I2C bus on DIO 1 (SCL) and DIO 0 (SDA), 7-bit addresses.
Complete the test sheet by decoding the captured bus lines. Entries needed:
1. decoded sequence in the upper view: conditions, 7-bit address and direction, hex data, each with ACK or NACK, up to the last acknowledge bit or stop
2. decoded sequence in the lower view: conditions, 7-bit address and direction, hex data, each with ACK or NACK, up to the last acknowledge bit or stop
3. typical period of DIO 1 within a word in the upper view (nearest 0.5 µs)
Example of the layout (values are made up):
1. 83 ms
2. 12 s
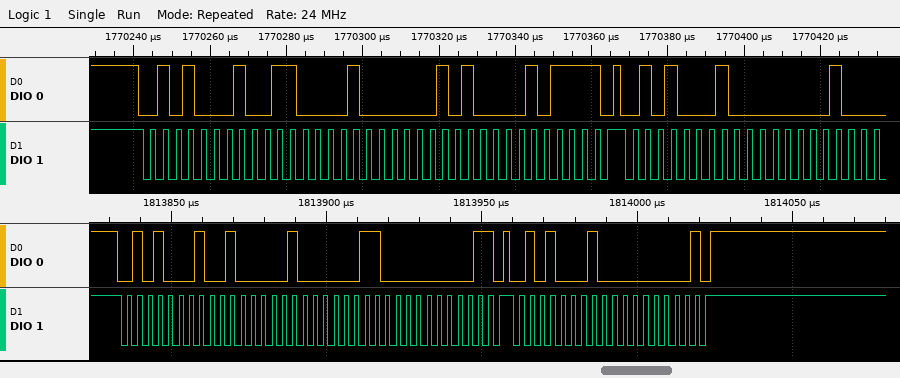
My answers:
1. start, address 28 read ACK, 61 ACK, 05 ACK, 17 NACK, stop, start, address 28 read ACK, 01 ACK
2. start, address 28 read ACK, 41 ACK, 06 ACK, 01 NACK, stop, start, address 28 read ACK, 00 NACK, stop
3. 3.5 µs
